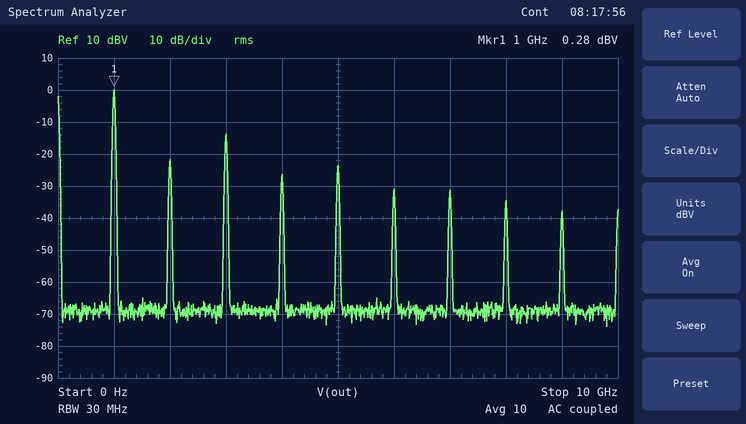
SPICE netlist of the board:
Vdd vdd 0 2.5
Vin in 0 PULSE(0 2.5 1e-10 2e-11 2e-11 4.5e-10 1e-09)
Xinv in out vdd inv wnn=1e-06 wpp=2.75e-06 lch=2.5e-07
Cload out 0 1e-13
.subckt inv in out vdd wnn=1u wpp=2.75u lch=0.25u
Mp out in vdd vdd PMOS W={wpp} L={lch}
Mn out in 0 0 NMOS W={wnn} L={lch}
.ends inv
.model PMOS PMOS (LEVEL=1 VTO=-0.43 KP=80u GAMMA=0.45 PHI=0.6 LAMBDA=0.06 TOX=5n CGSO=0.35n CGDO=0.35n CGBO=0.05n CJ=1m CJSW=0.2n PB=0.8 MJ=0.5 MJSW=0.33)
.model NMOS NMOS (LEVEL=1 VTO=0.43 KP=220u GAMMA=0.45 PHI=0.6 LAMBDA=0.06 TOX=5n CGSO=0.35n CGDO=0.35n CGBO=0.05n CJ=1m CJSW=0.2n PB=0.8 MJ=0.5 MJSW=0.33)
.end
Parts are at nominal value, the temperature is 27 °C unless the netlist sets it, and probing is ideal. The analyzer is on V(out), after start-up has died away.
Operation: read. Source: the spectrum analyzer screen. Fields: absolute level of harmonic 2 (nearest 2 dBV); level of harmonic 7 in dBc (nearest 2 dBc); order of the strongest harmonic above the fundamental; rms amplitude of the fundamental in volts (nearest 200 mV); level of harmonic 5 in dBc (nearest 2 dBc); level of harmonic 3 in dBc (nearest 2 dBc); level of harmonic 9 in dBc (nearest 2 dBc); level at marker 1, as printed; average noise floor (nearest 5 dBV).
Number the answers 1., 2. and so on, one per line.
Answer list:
1. -22 dBV
2. -32 dBc
3. 3
4. 1.0 V
5. -24 dBc
6. -14 dBc
7. -38 dBc
8. 0.28 dBV
9. -70 dBV
